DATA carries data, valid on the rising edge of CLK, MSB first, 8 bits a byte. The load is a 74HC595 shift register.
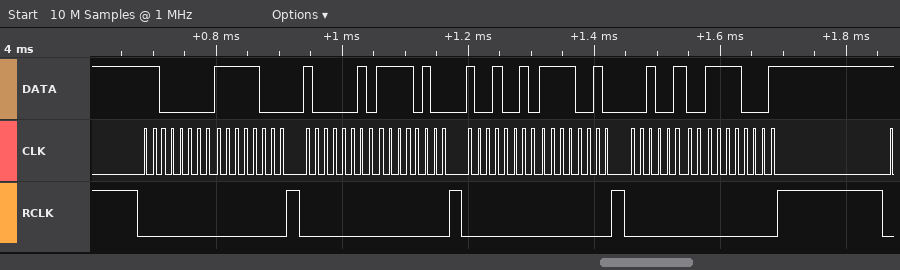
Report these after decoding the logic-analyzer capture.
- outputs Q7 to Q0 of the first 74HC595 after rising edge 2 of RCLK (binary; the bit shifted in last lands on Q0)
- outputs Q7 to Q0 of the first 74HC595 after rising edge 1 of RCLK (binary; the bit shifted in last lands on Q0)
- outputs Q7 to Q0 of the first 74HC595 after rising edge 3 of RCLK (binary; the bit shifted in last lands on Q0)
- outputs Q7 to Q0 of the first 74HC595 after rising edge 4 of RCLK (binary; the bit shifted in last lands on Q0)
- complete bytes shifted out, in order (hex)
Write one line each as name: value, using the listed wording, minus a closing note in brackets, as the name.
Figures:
outputs Q7 to Q0 of the first 74HC595 after rising edge 2 of RCLK: 11110100
outputs Q7 to Q0 of the first 74HC595 after rising edge 1 of RCLK: 11111000
outputs Q7 to Q0 of the first 74HC595 after rising edge 3 of RCLK: 11110010
outputs Q7 to Q0 of the first 74HC595 after rising edge 4 of RCLK: 11110001
complete bytes shifted out, in order: 0xC0 0xF8 0x82 0xF4 0x92 0xF2 0x24 0xF1
